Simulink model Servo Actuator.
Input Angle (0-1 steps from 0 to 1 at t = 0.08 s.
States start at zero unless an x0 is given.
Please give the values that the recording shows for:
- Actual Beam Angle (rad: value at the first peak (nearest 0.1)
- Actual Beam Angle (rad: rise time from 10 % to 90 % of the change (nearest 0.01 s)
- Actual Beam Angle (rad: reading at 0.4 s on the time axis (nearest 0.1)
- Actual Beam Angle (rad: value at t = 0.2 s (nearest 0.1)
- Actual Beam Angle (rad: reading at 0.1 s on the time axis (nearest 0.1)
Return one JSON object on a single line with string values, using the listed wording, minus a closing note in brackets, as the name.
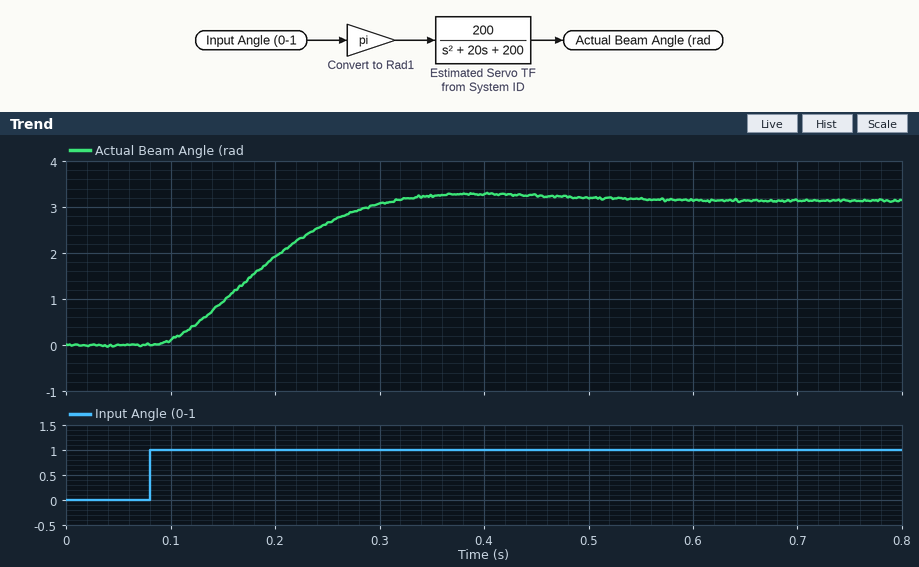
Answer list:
{"Actual Beam Angle (rad: value at the first peak": "3.3", "Actual Beam Angle (rad: rise time from 10 % to 90 % of the change": "0.15 s", "Actual Beam Angle (rad: reading at 0.4 s on the time axis": "3.3", "Actual Beam Angle (rad: value at t = 0.2 s": "1.9", "Actual Beam Angle (rad: reading at 0.1 s on the time axis": "0.1"}
